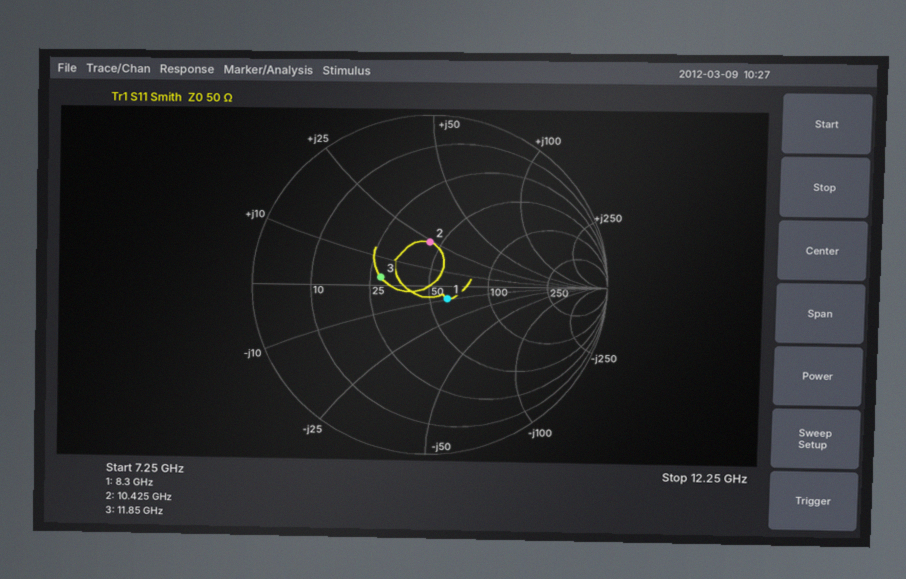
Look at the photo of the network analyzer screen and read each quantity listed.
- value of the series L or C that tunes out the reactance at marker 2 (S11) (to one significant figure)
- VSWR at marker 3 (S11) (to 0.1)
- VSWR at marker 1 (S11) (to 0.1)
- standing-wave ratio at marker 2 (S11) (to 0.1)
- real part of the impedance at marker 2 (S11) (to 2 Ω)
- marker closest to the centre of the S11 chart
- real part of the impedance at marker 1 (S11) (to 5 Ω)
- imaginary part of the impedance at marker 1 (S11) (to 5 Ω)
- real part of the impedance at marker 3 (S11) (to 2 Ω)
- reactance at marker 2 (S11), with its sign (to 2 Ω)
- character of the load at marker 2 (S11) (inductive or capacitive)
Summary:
600 fF
1.8
1.3
1.7
44 Ω
marker 1
60 Ω
-10 Ω
28 Ω
+24 Ω
inductive
